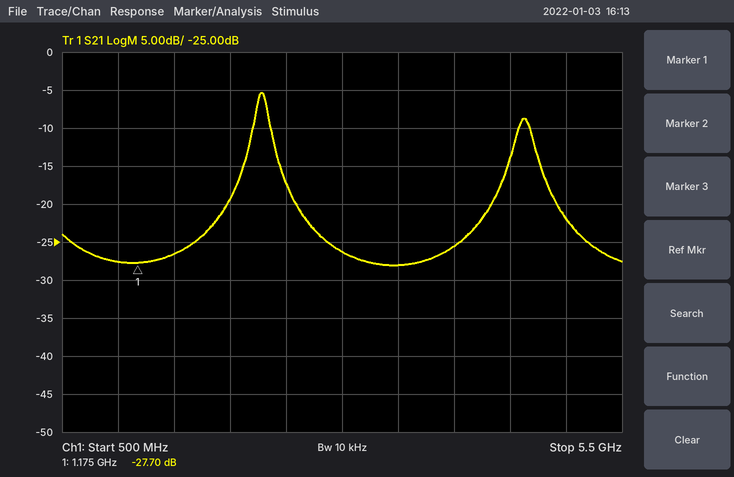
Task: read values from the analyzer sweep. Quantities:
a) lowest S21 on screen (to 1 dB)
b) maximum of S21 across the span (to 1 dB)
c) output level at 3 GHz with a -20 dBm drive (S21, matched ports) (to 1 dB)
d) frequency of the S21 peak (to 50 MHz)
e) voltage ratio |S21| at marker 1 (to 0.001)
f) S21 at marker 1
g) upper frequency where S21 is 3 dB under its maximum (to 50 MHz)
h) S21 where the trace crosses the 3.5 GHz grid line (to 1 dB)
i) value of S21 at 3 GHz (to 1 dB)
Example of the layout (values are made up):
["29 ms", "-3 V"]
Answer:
["-28 dB", "-5 dB", "-46 dBm", "2.30 GHz", "0.041", "-27.70 dB", "2.35 GHz", "-28 dB", "-26 dB"]
